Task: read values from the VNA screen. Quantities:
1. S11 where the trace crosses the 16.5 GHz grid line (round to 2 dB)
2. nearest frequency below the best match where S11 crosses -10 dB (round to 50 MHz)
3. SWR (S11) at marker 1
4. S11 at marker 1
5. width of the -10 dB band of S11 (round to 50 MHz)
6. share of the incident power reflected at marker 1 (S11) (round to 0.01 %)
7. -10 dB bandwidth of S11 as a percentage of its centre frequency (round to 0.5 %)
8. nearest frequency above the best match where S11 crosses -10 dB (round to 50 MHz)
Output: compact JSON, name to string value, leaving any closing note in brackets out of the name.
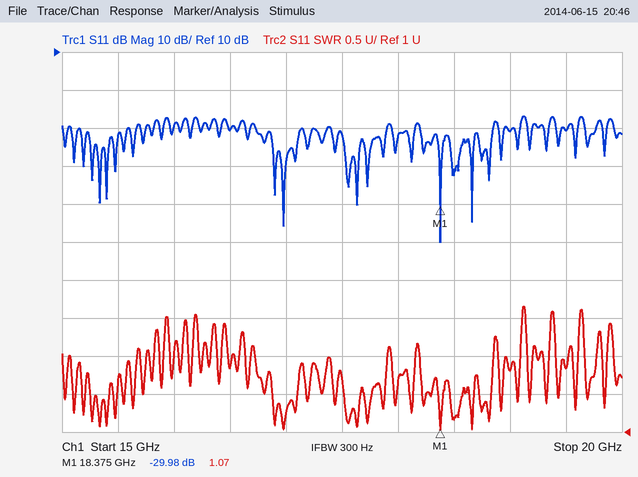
{"S11 where the trace crosses the 16.5 GHz grid line": "-10 dB", "nearest frequency below the best match where S11 crosses -10 dB": "18.20 GHz", "SWR (S11) at marker 1": "1.07", "S11 at marker 1": "-29.98 dB", "width of the -10 dB band of S11": "650 MHz", "share of the incident power reflected at marker 1 (S11)": "0.10 %", "-10 dB bandwidth of S11 as a percentage of its centre frequency": "3.5 %", "nearest frequency above the best match where S11 crosses -10 dB": "18.85 GHz"}
